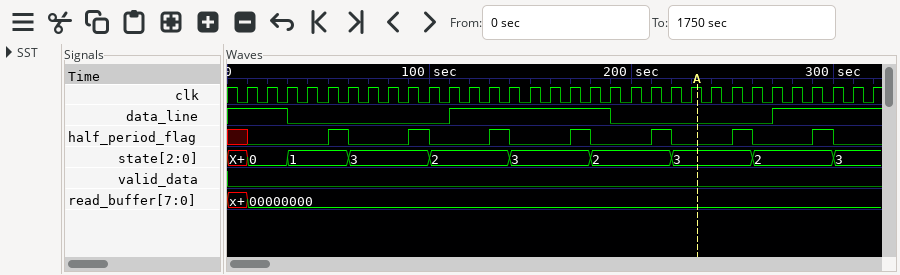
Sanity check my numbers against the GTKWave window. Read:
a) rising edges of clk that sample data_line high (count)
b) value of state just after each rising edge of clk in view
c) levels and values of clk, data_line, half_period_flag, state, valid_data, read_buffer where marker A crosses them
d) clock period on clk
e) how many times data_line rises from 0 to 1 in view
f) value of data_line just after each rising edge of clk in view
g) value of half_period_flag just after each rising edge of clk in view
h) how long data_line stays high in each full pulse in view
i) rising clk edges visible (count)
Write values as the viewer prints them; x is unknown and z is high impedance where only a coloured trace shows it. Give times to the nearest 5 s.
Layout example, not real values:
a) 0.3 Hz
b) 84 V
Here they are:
a) 16
b) 0, 0, 1, 1, 1, 3, 3, 3, 3, 2, 2, 2, 2, 3, 3, 3, 3, 2, 2, 2, 2, 3, 3, 3, 3, 2, 2, 2, 2, 3, 3, 3
c) clk=1, data_line=0, half_period_flag=0, state=3, valid_data=0, read_buffer=00000000
d) 10 s
e) 2
f) 1 1 0 0 0 0 0 0 0 0 1 1 1 1 1 1 1 1 0 0 0 0 0 0 0 0 1 1 1 1 1 1
g) 0 0 0 0 1 0 0 0 1 0 0 0 1 0 0 0 1 0 0 0 1 0 0 0 1 0 0 0 1 0 0 0
h) 80 s
i) 32
